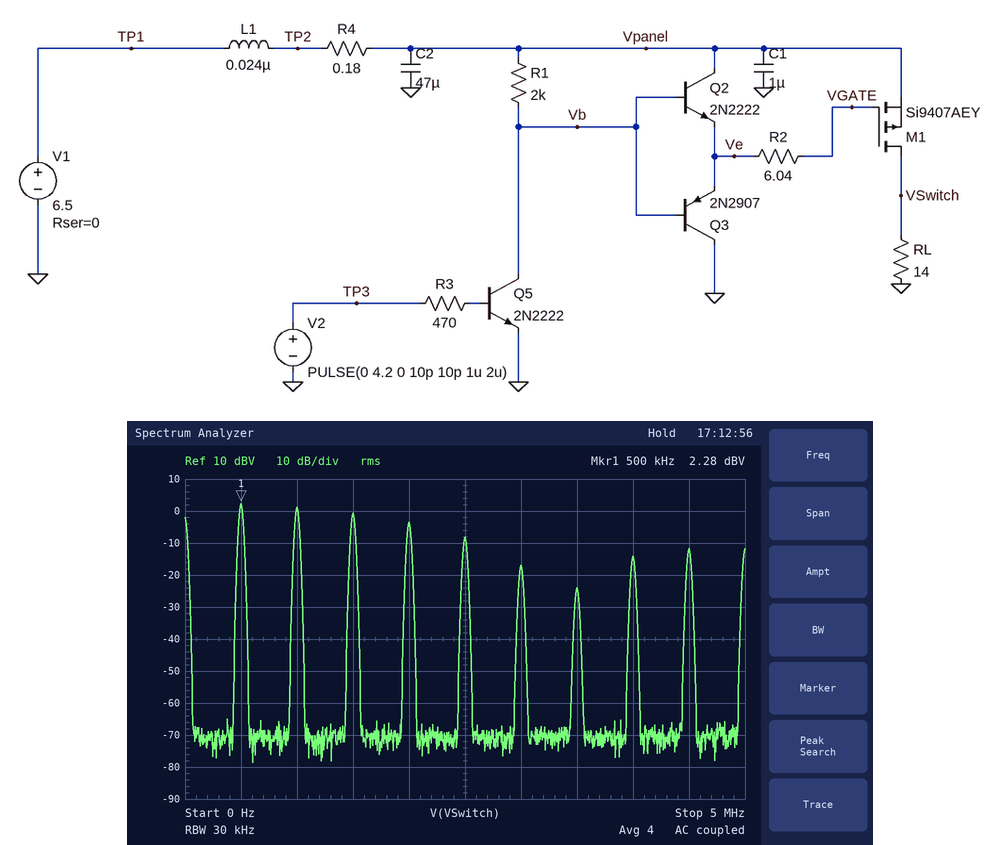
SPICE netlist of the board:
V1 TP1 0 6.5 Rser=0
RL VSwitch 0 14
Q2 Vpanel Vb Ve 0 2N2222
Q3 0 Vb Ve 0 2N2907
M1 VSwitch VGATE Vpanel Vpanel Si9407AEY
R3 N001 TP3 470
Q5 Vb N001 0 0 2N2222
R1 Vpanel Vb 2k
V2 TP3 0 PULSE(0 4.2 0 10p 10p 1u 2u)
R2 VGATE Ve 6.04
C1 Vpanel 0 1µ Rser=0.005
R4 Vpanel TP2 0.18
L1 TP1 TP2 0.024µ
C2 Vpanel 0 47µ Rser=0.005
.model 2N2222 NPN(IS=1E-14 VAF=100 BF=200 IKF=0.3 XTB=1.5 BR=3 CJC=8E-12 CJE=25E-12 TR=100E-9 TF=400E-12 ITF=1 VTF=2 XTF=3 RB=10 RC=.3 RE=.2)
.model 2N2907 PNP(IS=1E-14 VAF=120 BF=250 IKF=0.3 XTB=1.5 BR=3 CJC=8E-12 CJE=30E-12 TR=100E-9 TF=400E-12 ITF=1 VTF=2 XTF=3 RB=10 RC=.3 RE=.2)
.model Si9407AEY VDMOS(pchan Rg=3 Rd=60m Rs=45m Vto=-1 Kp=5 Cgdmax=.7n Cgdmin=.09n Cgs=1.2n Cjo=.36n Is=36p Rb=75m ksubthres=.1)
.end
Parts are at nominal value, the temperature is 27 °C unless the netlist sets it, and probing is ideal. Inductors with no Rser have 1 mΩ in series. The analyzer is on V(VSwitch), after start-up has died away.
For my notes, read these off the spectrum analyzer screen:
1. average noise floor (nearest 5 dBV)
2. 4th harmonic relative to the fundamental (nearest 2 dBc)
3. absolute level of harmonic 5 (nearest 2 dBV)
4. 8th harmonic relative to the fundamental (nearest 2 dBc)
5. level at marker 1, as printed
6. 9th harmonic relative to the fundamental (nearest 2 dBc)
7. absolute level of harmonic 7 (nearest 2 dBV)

-70 dBV
-6 dBc
-8 dBV
-16 dBc
2.28 dBV
-14 dBc
-24 dBV
